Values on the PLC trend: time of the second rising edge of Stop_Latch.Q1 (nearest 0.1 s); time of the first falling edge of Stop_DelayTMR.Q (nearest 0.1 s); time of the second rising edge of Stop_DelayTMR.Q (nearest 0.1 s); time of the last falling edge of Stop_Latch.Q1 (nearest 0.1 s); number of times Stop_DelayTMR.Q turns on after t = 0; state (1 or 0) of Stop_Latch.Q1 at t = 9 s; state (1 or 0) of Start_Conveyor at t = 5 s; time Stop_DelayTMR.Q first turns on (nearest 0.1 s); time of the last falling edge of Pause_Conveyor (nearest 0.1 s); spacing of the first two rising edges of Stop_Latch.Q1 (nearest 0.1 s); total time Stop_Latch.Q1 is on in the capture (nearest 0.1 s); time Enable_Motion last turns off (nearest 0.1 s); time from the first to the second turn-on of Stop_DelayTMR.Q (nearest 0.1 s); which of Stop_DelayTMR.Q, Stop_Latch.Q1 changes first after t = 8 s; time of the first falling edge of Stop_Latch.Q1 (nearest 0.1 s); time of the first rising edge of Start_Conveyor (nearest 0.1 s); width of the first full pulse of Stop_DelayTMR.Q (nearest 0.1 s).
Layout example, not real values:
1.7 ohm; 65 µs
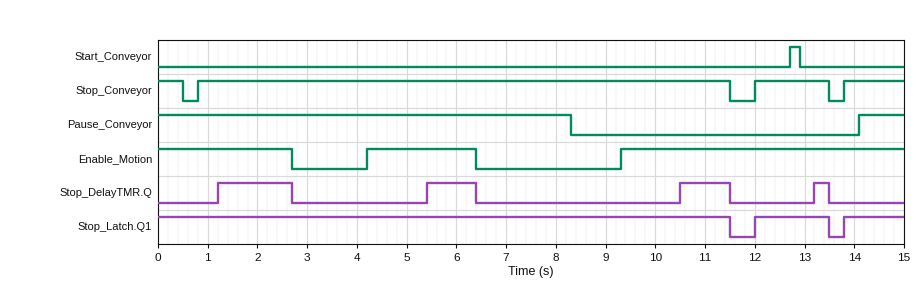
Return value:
13.8 s; 2.7 s; 5.4 s; 13.5 s; 4; 1; 0; 1.2 s; 8.3 s; 1.8 s; 14.2 s; 6.4 s; 4.2 s; Stop_DelayTMR.Q; 11.5 s; 12.7 s; 1.5 s
